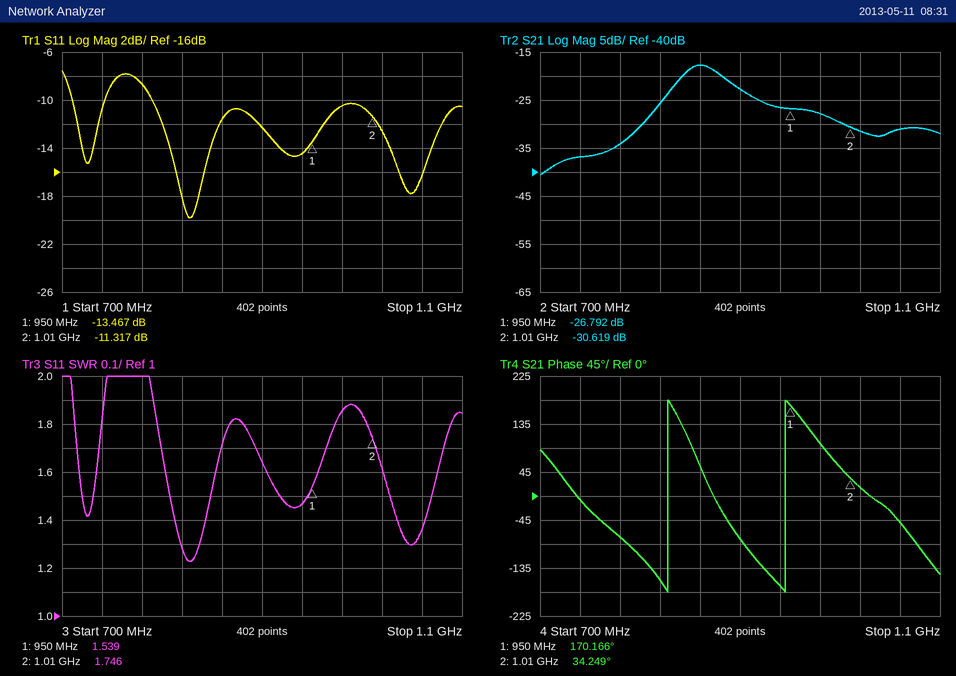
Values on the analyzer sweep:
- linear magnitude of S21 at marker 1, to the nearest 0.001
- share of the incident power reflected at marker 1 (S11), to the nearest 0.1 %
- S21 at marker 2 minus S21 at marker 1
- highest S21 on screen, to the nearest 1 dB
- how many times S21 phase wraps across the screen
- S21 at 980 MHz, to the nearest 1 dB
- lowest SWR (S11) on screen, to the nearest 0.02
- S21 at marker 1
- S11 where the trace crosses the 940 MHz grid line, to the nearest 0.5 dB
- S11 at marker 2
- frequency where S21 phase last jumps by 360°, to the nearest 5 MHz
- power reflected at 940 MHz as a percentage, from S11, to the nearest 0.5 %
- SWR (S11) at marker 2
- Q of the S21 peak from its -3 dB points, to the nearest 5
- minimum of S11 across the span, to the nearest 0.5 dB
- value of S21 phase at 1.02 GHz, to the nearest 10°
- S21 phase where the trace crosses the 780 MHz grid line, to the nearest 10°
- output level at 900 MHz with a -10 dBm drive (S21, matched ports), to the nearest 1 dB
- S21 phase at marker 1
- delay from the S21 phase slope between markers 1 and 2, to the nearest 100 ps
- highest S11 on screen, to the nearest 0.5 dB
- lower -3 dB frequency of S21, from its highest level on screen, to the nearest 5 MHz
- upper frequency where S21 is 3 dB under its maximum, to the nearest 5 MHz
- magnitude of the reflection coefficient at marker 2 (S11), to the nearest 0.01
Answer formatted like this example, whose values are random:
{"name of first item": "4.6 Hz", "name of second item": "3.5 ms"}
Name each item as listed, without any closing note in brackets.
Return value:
{"linear magnitude of S21 at marker 1, to the nearest 0.001": "0.046", "share of the incident power reflected at marker 1 (S11), to the nearest 0.1 %": "4.5 %", "S21 at marker 2 minus S21 at marker 1": "-3.827 dB", "highest S21 on screen, to the nearest 1 dB": "-18 dB", "how many times S21 phase wraps across the screen": "2", "S21 at 980 MHz, to the nearest 1 dB": "-28 dB", "lowest SWR (S11) on screen, to the nearest 0.02": "1.22", "S21 at marker 1": "-26.792 dB", "S11 where the trace crosses the 940 MHz grid line, to the nearest 0.5 dB": "-14.5 dB", "S11 at marker 2": "-11.317 dB", "frequency where S21 phase last jumps by 360°, to the nearest 5 MHz": "945 MHz", "power reflected at 940 MHz as a percentage, from S11, to the nearest 0.5 %": "3.5 %", "SWR (S11) at marker 2": "1.746", "Q of the S21 peak from its -3 dB points, to the nearest 5": "20", "minimum of S11 across the span, to the nearest 0.5 dB": "-20.0 dB", "value of S21 phase at 1.02 GHz, to the nearest 10°": "20°", "S21 phase where the trace crosses the 780 MHz grid line, to the nearest 10°": "-80°", "output level at 900 MHz with a -10 dBm drive (S21, matched ports), to the nearest 1 dB": "-33 dBm", "S21 phase at marker 1": "170.166°", "delay from the S21 phase slope between markers 1 and 2, to the nearest 100 ps": "6.3 ns", "highest S11 on screen, to the nearest 0.5 dB": "-7.5 dB", "lower -3 dB frequency of S21, from its highest level on screen, to the nearest 5 MHz": "840 MHz", "upper frequency where S21 is 3 dB under its maximum, to the nearest 5 MHz": "885 MHz", "magnitude of the reflection coefficient at marker 2 (S11), to the nearest 0.01": "0.27"}
